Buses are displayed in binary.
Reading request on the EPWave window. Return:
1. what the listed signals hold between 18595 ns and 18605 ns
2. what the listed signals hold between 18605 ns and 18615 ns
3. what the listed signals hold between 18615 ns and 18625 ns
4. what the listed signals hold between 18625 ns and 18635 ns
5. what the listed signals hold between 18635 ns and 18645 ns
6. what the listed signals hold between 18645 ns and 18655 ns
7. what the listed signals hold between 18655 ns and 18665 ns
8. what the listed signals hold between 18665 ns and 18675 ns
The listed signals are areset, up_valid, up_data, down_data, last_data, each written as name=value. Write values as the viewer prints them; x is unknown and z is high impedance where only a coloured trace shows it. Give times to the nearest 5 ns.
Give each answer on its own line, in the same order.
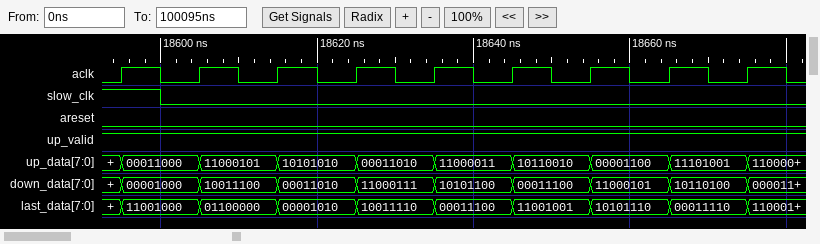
areset=0, up_valid=1, up_data=00011000, down_data=00001000, last_data=11001000
areset=0, up_valid=1, up_data=11000101, down_data=10011100, last_data=01100000
areset=0, up_valid=1, up_data=10101010, down_data=00011010, last_data=00001010
areset=0, up_valid=1, up_data=00011010, down_data=11000111, last_data=10011110
areset=0, up_valid=1, up_data=11000011, down_data=10101100, last_data=00011100
areset=0, up_valid=1, up_data=10110010, down_data=00011100, last_data=11001001
areset=0, up_valid=1, up_data=00001100, down_data=11000101, last_data=10101110
areset=0, up_valid=1, up_data=11101001, down_data=10110100, last_data=00011110
